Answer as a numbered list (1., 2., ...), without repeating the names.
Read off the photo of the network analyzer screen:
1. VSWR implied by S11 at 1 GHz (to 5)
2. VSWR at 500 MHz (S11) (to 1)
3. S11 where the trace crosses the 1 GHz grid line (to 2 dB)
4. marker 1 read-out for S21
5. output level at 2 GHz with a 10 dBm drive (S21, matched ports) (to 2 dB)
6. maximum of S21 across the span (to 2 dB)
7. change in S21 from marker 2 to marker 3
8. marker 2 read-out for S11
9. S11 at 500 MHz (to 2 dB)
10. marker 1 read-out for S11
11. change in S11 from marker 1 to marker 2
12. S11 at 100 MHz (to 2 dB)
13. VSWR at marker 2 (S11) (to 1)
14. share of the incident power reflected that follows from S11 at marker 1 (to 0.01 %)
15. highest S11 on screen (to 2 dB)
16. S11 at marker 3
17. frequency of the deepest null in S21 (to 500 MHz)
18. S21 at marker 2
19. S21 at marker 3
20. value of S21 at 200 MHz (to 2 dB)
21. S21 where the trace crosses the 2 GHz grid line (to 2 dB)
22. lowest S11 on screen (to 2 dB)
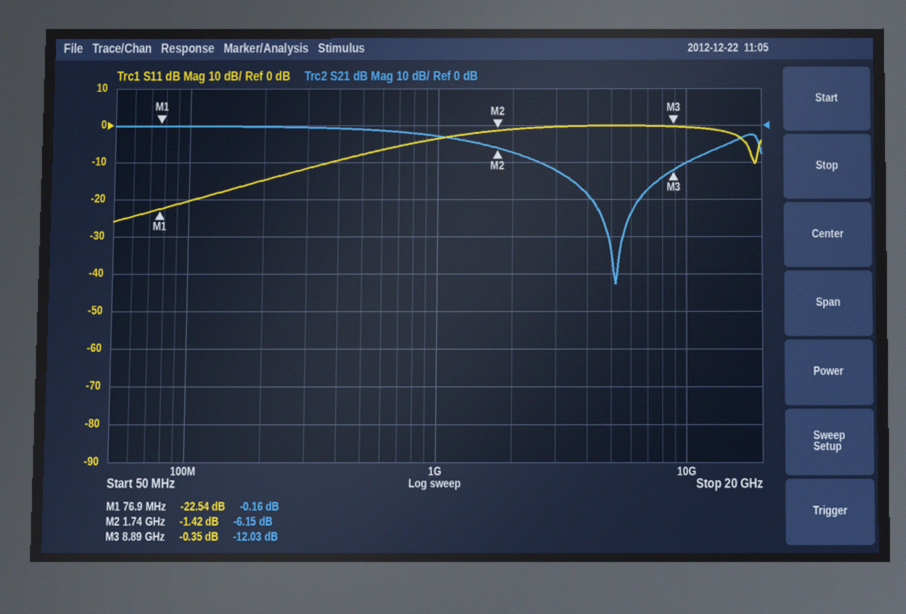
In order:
1. 5
2. 2
3. -4 dB
4. -0.16 dB
5. 2 dBm
6. 0 dB
7. -5.88 dB
8. -1.42 dB
9. -8 dB
10. -22.54 dB
11. 21.12 dB
12. -20 dB
13. 12
14. 0.56 %
15. 0 dB
16. -0.35 dB
17. 5.0 GHz
18. -6.15 dB
19. -12.03 dB
20. 0 dB
21. -8 dB
22. -26 dB
